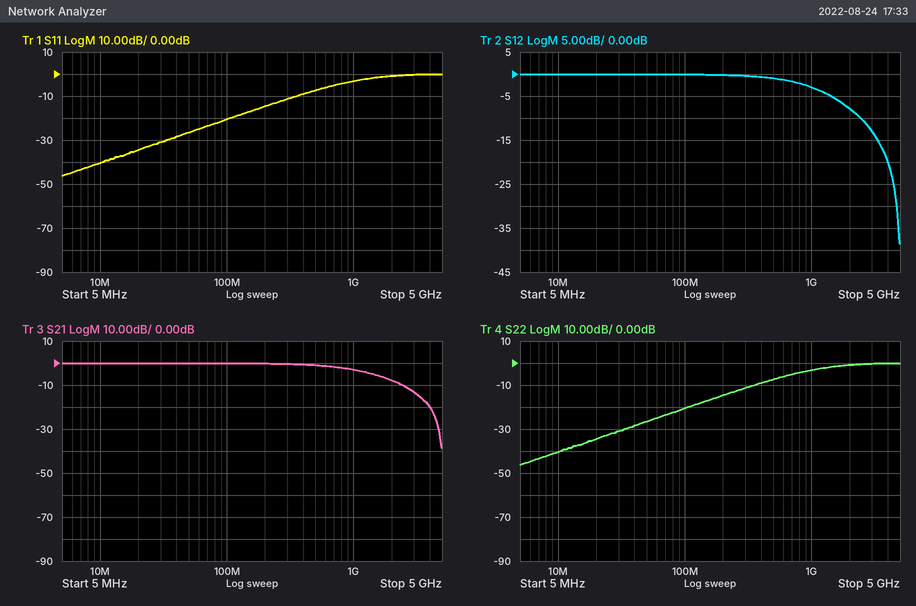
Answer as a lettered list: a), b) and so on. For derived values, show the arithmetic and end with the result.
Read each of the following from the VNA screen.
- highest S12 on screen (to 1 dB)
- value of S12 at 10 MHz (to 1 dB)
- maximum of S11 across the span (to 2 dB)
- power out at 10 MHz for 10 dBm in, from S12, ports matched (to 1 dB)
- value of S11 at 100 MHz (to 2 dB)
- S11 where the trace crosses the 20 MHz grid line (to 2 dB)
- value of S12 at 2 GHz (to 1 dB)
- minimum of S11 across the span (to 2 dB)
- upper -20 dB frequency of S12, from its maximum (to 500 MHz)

a) 0 dB
b) 0 dB
c) 0 dB
d) 10 dBm + (0 dB) = 10 dBm
e) -20 dB
f) -34 dB
g) -8 dB
h) -46 dB
i) 4.0 GHz
